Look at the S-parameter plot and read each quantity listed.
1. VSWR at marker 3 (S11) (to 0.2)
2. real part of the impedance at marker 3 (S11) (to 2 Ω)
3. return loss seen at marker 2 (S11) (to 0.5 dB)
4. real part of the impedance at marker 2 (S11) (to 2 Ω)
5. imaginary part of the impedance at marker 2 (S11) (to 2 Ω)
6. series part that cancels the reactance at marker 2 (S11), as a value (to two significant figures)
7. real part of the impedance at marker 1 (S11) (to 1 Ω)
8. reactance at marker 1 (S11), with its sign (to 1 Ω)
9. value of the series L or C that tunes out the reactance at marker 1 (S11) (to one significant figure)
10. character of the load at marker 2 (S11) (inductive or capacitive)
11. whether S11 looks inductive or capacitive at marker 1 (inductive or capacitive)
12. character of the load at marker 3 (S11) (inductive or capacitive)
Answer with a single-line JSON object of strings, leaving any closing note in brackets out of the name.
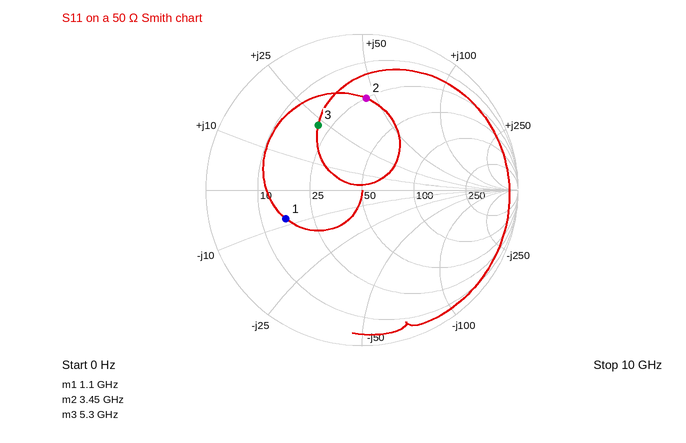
{"VSWR at marker 3 (S11)": "3.0", "real part of the impedance at marker 3 (S11)": "20 Ω", "return loss seen at marker 2 (S11)": "4.5 dB", "real part of the impedance at marker 2 (S11)": "26 Ω", "imaginary part of the impedance at marker 2 (S11)": "+46 Ω", "series part that cancels the reactance at marker 2 (S11), as a value": "1.0 pF", "real part of the impedance at marker 1 (S11)": "16 Ω", "reactance at marker 1 (S11), with its sign": "-8 Ω", "value of the series L or C that tunes out the reactance at marker 1 (S11)": "1 nH", "character of the load at marker 2 (S11)": "inductive", "whether S11 looks inductive or capacitive at marker 1": "capacitive", "character of the load at marker 3 (S11)": "inductive"}
